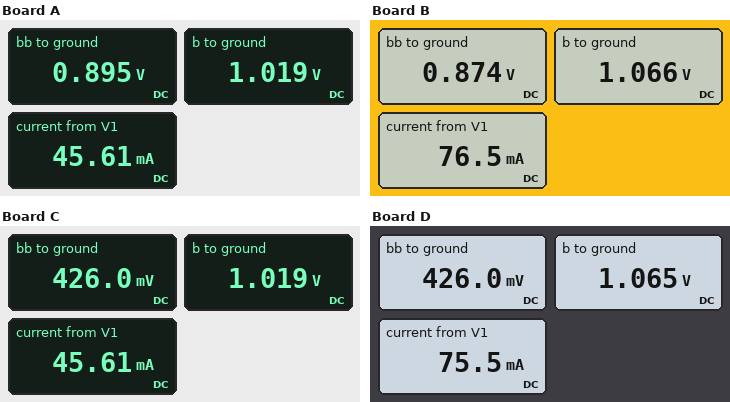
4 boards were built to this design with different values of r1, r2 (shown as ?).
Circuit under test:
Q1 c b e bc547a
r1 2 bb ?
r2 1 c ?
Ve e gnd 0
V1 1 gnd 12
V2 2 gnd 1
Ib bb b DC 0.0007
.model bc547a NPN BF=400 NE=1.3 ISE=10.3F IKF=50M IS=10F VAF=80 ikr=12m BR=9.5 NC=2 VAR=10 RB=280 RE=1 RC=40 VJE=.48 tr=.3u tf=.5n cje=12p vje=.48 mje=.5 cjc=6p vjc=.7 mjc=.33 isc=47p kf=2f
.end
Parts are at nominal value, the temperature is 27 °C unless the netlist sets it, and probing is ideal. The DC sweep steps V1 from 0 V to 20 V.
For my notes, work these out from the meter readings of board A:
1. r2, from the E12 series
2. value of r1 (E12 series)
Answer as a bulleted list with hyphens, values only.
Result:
- 220 Ω
- 150 Ω
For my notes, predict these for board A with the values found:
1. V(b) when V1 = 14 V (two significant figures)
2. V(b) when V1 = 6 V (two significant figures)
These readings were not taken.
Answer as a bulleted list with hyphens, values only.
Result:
- 1.0 V
- 980 mV
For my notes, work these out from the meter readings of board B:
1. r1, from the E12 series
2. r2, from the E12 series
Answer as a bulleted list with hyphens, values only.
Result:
- 180 Ω
- 68 Ω
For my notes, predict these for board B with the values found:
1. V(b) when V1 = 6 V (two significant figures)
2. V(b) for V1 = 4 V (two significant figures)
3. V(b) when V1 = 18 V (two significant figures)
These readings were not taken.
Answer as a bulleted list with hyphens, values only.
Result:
- 1.0 V
- 1.0 V
- 1.1 V
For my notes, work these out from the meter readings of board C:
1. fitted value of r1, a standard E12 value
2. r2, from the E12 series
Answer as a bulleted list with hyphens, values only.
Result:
- 820 Ω
- 220 Ω
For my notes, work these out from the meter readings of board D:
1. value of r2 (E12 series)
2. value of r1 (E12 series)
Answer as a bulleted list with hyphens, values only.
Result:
- 82 Ω
- 820 Ω
